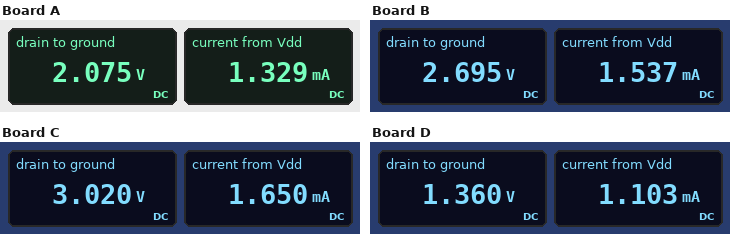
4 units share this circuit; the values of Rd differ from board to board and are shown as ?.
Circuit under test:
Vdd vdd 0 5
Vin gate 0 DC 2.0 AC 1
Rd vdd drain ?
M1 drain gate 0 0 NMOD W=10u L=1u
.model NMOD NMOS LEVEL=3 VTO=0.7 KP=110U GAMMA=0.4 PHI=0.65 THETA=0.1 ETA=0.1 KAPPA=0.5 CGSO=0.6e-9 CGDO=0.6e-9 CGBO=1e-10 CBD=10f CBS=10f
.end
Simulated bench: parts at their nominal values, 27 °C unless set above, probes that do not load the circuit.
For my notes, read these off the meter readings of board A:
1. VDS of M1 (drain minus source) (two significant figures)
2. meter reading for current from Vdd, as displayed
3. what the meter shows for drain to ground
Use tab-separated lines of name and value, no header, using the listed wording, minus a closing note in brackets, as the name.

VDS of M1 (drain minus source)	2.1 V
meter reading for current from Vdd, as displayed	1.329 mA
what the meter shows for drain to ground	2.075 V
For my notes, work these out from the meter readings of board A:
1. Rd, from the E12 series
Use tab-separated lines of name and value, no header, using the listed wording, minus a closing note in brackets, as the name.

Rd, from the E12 series	2.2 kΩ
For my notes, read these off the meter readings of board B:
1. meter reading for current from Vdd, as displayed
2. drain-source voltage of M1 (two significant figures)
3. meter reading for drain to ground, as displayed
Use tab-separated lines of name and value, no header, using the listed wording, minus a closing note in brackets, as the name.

meter reading for current from Vdd, as displayed	1.537 mA
drain-source voltage of M1	2.7 V
meter reading for drain to ground, as displayed	2.695 V
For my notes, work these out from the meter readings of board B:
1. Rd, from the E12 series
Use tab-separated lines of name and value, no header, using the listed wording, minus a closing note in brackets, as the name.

Rd, from the E12 series	1.5 kΩ
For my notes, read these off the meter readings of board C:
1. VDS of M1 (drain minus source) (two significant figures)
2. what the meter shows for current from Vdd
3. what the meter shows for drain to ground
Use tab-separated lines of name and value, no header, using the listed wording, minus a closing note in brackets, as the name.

VDS of M1 (drain minus source)	3.0 V
what the meter shows for current from Vdd	1.650 mA
what the meter shows for drain to ground	3.020 V
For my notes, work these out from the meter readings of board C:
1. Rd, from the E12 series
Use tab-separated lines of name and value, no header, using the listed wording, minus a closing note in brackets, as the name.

Rd, from the E12 series	1.2 kΩ
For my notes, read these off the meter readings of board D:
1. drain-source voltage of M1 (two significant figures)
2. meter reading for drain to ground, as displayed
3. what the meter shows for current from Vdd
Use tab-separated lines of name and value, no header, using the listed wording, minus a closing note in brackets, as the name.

drain-source voltage of M1	1.4 V
meter reading for drain to ground, as displayed	1.360 V
what the meter shows for current from Vdd	1.103 mA
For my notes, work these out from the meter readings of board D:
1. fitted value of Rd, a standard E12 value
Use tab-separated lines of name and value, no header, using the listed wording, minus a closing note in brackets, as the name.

fitted value of Rd, a standard E12 value	3.3 kΩ
